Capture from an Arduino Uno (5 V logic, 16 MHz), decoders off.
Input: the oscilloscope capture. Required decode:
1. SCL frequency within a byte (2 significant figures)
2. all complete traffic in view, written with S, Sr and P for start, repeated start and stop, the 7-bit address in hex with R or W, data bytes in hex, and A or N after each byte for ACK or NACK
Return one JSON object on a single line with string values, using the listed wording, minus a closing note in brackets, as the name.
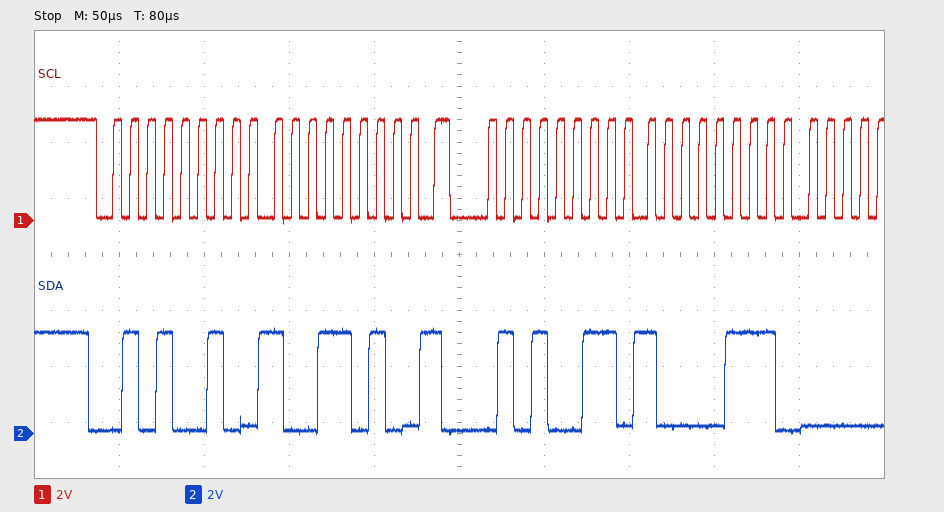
{"SCL frequency within a byte": "100 kHz", "all complete traffic in view, written with S, Sr and P for start, repeated start and stop, the 7-bit address in hex with R or W, data bytes in hex, and A or N after each byte for ACK or NACK": "S 29W A 9A A Sr 29R A 87 A"}
